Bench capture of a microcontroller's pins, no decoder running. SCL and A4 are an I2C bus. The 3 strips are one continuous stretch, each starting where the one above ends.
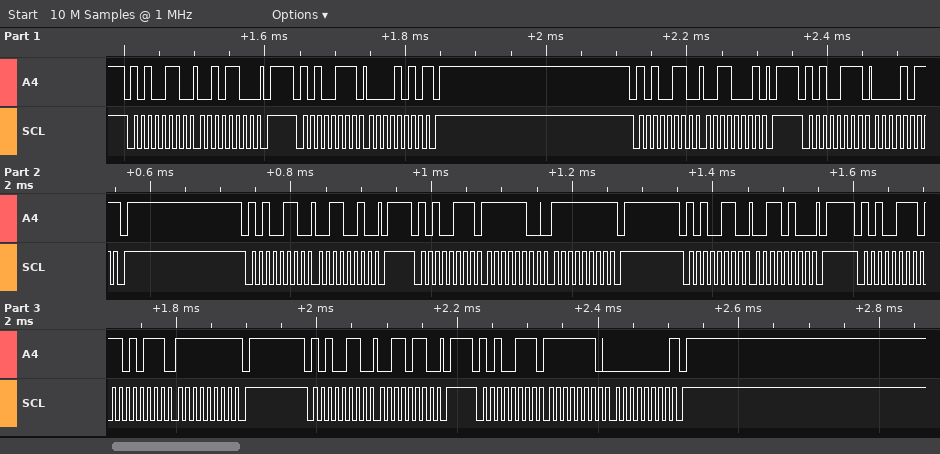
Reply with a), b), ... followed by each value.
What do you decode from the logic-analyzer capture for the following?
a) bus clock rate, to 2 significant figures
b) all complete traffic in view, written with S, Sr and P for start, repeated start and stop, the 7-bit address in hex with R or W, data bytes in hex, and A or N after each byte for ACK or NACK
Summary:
a) 100 kHz
b) S 53W A 2C A P S 53R A 0A N P S 53W A 31 A P S 53R A 0B N P S 53W A 32 A P S 53R A FC A FF N P S 53W A 34 A P S 53R A D7 A FF N P S 53W A 36 A P S 53R A FE A 00 N P
